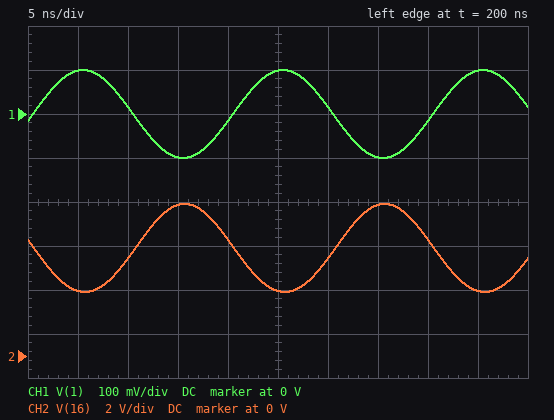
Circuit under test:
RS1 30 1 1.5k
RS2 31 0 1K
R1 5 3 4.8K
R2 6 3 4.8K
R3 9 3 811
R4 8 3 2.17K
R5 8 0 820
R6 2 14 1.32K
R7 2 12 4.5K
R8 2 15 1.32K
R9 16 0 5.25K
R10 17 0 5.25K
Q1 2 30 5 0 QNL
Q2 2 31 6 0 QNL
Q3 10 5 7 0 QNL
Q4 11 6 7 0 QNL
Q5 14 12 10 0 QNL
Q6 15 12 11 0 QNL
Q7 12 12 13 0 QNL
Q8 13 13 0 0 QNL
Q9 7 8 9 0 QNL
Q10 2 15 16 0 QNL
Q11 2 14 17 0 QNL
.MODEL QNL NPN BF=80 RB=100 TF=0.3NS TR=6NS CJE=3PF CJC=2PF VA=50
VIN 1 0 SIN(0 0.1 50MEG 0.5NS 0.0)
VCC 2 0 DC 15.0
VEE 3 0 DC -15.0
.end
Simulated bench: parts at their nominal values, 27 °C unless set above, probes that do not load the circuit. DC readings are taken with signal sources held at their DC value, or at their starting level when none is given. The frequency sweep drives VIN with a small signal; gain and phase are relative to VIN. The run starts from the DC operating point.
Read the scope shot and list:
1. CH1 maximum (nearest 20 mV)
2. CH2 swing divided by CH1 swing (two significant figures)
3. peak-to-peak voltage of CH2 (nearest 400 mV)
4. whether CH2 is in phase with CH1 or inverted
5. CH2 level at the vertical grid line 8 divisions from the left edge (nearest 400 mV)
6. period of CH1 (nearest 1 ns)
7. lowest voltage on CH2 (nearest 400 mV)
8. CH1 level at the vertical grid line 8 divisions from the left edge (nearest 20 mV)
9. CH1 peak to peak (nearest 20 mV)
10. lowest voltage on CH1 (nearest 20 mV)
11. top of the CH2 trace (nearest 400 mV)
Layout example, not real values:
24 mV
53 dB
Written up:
100 mV
20
4.0 V
inverted
5.2 V
20 ns
2.8 V
-20 mV
200 mV
-100 mV
6.8 V
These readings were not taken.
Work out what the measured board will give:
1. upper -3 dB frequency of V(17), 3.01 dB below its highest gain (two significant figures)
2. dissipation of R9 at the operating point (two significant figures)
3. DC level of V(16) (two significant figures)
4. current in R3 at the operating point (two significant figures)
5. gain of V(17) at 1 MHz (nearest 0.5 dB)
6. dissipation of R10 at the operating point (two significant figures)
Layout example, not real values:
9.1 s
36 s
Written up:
23 MHz
4.4 mW
4.8 V
12 mA
40.5 dB
12 mW
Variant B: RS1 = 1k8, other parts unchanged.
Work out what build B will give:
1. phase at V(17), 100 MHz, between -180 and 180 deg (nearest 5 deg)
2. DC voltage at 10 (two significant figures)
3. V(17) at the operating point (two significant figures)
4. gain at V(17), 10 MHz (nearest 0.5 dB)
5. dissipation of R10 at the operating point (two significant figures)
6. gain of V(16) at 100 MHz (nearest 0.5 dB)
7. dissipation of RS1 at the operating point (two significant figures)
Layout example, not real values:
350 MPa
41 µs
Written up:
-55 deg
800 mV
8.9 V
40.0 dB
15 mW
8.5 dB
1.5 µW
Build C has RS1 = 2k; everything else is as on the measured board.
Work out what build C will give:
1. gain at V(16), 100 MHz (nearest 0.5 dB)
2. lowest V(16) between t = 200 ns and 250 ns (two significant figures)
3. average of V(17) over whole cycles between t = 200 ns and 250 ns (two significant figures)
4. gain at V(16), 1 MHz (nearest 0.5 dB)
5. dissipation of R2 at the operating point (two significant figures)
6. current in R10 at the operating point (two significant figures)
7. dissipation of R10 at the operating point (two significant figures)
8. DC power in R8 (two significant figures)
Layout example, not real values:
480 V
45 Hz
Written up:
7.5 dB
1.9 V
9.3 V
39.5 dB
42 mW
1.8 mA
17 mW
90 mW
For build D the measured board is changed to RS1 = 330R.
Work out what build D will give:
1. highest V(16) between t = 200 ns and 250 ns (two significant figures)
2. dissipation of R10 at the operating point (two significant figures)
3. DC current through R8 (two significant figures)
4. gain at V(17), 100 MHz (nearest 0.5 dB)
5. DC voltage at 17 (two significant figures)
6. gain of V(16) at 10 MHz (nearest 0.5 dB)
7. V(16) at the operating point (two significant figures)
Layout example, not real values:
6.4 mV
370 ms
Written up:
11 V
3.5 mW
4.3 mA
15.0 dB
4.3 V
40.0 dB
8.5 V
